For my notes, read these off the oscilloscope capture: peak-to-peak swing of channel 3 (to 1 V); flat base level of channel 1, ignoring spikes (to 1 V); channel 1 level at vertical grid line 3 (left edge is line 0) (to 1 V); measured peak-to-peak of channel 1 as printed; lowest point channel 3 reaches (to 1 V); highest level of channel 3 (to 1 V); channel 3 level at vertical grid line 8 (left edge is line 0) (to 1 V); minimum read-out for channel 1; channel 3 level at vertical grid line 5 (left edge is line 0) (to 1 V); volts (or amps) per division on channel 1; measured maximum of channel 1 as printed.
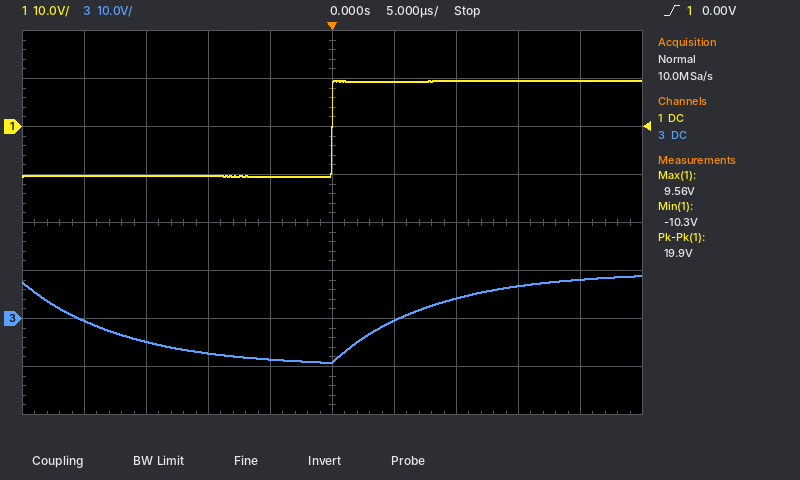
18 V
-10 V
-10 V
19.9 V
-9 V
9 V
7 V
-10.3 V
-9 V
10 V
9.56 V
